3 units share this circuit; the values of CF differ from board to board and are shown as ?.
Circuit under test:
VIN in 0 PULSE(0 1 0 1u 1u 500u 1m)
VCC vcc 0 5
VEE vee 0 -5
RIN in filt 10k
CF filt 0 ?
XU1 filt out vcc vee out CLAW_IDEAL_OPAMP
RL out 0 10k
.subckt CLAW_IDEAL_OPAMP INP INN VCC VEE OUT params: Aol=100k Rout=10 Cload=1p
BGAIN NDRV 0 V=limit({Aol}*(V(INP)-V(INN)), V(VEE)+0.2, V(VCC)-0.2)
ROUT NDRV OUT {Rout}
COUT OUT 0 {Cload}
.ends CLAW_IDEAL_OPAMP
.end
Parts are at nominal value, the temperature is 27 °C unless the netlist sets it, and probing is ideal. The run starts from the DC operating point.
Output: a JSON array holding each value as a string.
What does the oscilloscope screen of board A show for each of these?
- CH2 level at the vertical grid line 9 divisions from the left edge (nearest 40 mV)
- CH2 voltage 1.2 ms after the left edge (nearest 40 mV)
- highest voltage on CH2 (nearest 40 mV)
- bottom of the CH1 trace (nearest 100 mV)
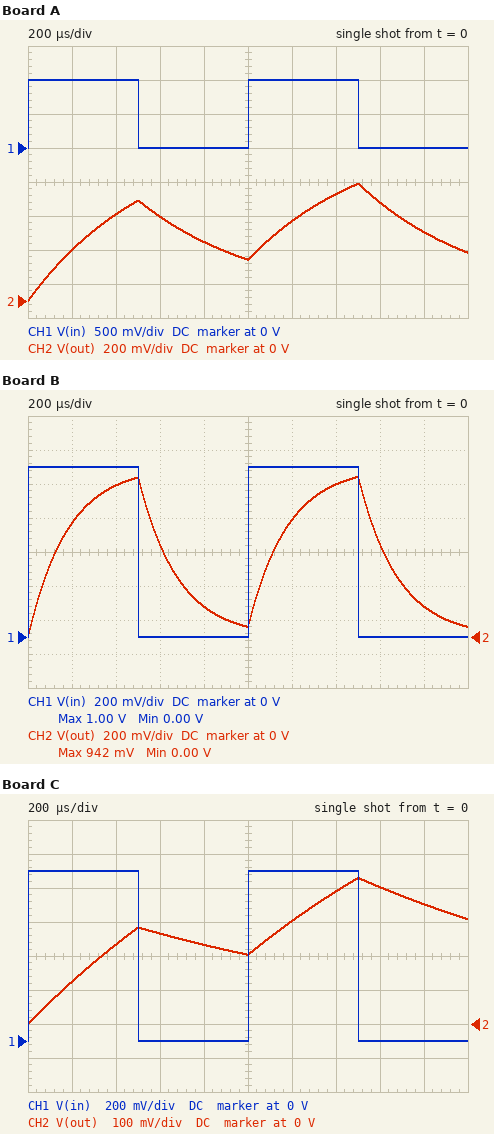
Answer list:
["400 mV", "480 mV", "680 mV", "0 V"]
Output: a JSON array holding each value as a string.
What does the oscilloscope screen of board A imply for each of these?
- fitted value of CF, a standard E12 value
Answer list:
["56 nF"]
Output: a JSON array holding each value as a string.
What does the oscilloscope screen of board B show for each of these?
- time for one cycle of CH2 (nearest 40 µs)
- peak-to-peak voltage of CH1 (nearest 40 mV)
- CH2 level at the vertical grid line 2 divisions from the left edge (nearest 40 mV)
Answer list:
["1.00 ms", "1.00 V", "880 mV"]
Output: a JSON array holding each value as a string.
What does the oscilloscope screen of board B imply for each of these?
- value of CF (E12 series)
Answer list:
["18 nF"]
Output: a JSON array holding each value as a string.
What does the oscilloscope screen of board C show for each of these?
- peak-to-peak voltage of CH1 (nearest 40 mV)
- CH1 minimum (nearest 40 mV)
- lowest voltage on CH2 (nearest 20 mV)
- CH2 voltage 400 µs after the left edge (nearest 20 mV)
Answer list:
["1.00 V", "0 V", "0 V", "240 mV"]
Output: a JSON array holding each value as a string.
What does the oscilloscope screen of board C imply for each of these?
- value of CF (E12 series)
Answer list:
["150 nF"]
